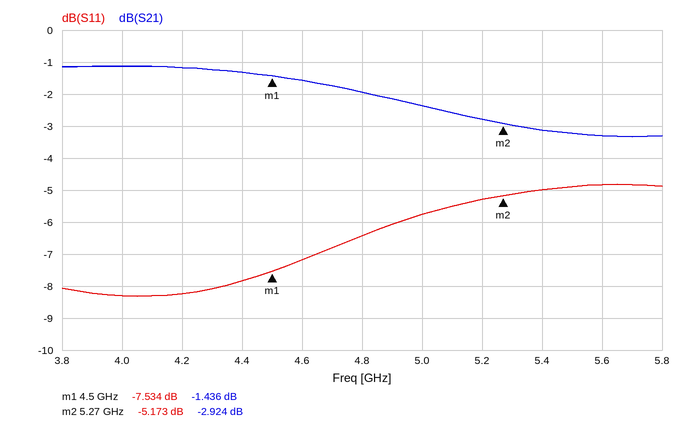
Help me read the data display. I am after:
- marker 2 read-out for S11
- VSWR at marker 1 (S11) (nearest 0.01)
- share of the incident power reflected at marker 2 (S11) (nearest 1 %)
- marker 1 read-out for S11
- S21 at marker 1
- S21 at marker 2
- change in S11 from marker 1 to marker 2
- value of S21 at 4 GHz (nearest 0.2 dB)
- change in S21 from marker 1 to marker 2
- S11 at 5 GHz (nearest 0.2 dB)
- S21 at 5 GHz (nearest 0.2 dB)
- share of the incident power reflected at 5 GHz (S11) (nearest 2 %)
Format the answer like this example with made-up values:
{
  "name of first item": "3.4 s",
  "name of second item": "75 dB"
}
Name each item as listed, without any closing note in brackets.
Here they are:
{
  "marker 2 read-out for S11": "-5.173 dB",
  "VSWR at marker 1 (S11)": "2.45",
  "share of the incident power reflected at marker 2 (S11)": "30 %",
  "marker 1 read-out for S11": "-7.534 dB",
  "S21 at marker 1": "-1.436 dB",
  "S21 at marker 2": "-2.924 dB",
  "change in S11 from marker 1 to marker 2": "2.361 dB",
  "value of S21 at 4 GHz": "-1.2 dB",
  "change in S21 from marker 1 to marker 2": "-1.488 dB",
  "S11 at 5 GHz": "-5.8 dB",
  "S21 at 5 GHz": "-2.4 dB",
  "share of the incident power reflected at 5 GHz (S11)": "26 %"
}
